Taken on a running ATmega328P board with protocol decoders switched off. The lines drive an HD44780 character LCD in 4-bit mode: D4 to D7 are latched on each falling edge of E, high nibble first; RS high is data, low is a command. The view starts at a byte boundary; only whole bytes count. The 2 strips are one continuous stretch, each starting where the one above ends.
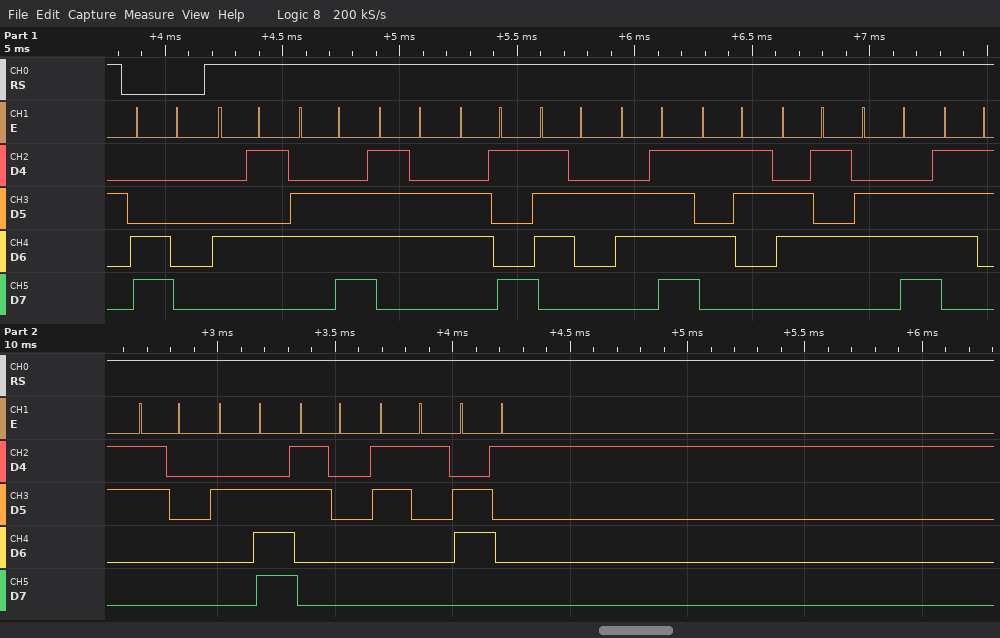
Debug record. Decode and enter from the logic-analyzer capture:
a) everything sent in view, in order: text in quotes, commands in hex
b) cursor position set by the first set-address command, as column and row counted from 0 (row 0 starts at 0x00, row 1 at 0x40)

0xC0 "EnviroSens0.01a"
column 0, row 1
